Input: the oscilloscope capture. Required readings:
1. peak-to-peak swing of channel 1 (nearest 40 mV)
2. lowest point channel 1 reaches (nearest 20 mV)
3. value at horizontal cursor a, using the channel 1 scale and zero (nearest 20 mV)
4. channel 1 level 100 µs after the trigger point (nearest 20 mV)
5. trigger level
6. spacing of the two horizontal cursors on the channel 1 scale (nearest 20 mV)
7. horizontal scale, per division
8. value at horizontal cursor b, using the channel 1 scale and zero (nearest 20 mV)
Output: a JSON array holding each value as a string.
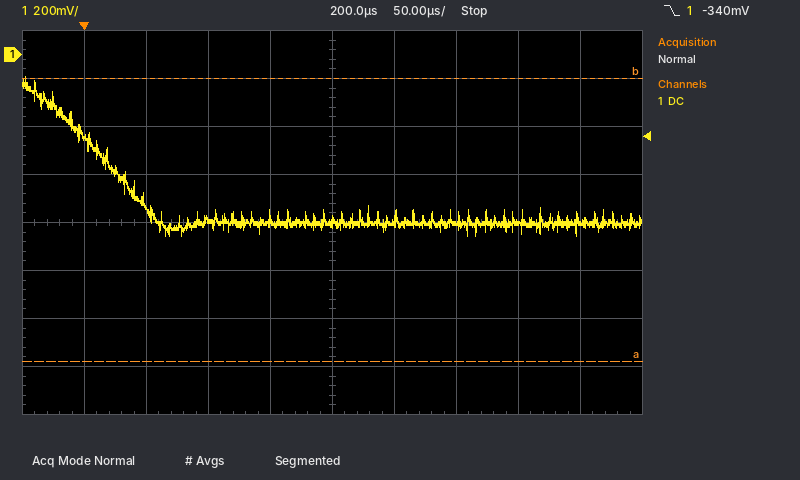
["680 mV", "-760 mV", "-1.28 V", "-680 mV", "-340 mV", "1.18 V", "50 µs", "-100 mV"]
